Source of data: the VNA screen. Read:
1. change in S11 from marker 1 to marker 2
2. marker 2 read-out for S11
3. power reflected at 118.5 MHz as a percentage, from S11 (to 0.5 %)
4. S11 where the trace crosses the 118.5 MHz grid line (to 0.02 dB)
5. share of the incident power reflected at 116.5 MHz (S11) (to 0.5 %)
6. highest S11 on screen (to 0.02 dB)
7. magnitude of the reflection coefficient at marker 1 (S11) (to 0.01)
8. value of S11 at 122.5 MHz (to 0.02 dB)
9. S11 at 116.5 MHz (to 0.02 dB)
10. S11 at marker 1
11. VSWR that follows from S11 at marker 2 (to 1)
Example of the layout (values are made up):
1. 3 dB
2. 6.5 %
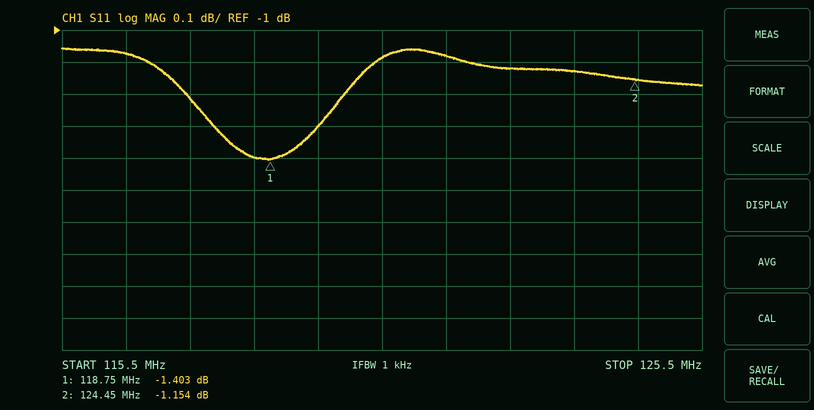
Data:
1. 0.249 dB
2. -1.154 dB
3. 72.5 %
4. -1.40 dB
5. 78.0 %
6. -1.06 dB
7. 0.85
8. -1.12 dB
9. -1.08 dB
10. -1.403 dB
11. 15
